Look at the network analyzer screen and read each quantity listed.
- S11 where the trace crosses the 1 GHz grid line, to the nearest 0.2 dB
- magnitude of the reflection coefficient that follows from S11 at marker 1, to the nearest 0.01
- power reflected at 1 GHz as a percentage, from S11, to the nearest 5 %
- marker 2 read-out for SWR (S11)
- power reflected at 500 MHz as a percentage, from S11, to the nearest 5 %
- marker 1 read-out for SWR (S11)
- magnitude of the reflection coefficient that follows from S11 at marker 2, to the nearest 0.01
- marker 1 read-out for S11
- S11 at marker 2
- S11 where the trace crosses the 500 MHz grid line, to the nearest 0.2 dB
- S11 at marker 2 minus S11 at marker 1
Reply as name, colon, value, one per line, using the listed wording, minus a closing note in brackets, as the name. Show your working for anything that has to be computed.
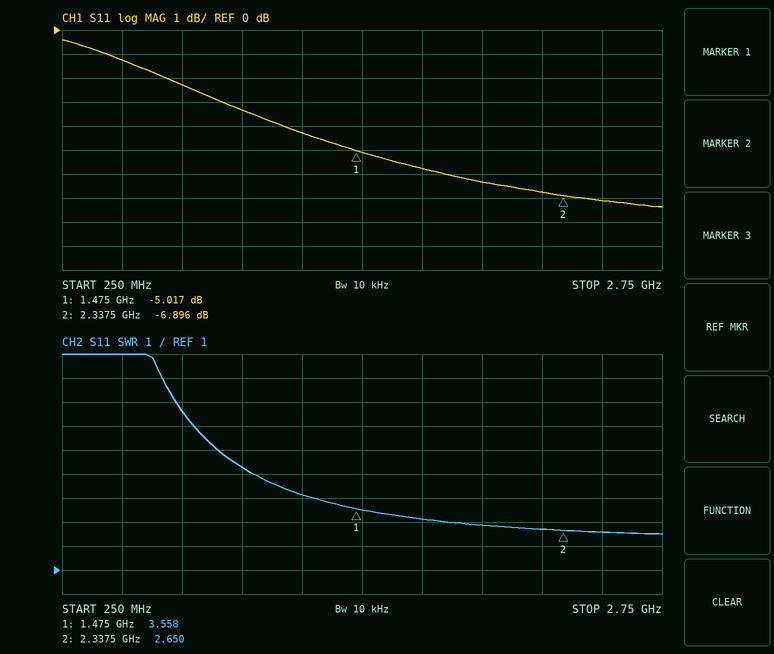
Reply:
S11 where the trace crosses the 1 GHz grid line, to the nearest 0.2 dB: -3.4 dB
magnitude of the reflection coefficient that follows from S11 at marker 1, to the nearest 0.01: 10^(-5.017/20) ≈ 0.56
power reflected at 1 GHz as a percentage, from S11, to the nearest 5 %: 10^(-3.4/10) ≈ 45.7 %, so 45 % to the nearest 5 %
marker 2 read-out for SWR: 2.650
power reflected at 500 MHz as a percentage, from S11, to the nearest 5 %: 10^(-1.2/10) ≈ 75.9 %, so 75 % to the nearest 5 %
marker 1 read-out for SWR: 3.558
magnitude of the reflection coefficient that follows from S11 at marker 2, to the nearest 0.01: 10^(-6.896/20) ≈ 0.45
marker 1 read-out for S11: -5.017 dB
S11 at marker 2: -6.896 dB
S11 where the trace crosses the 500 MHz grid line, to the nearest 0.2 dB: -1.2 dB
S11 at marker 2 minus S11 at marker 1: -6.896 − (-5.017) = -1.879 dB
